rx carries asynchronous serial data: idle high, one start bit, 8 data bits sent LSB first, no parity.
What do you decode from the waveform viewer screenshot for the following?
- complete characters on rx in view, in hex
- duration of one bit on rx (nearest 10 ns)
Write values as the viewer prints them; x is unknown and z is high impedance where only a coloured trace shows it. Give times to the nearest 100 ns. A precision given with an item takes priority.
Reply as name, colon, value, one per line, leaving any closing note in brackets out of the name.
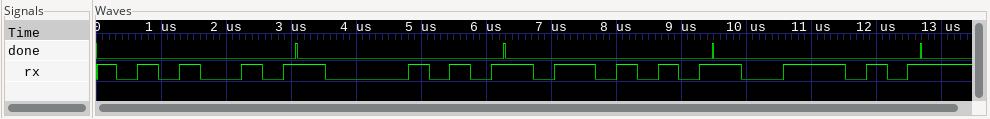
complete characters on rx in view, in hex: A5, A8, AB, AE
duration of one bit on rx: 320 ns
